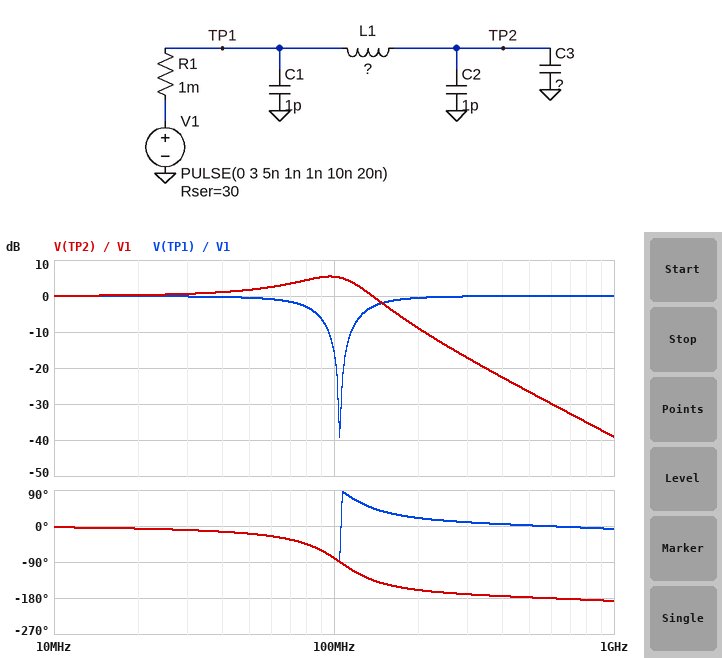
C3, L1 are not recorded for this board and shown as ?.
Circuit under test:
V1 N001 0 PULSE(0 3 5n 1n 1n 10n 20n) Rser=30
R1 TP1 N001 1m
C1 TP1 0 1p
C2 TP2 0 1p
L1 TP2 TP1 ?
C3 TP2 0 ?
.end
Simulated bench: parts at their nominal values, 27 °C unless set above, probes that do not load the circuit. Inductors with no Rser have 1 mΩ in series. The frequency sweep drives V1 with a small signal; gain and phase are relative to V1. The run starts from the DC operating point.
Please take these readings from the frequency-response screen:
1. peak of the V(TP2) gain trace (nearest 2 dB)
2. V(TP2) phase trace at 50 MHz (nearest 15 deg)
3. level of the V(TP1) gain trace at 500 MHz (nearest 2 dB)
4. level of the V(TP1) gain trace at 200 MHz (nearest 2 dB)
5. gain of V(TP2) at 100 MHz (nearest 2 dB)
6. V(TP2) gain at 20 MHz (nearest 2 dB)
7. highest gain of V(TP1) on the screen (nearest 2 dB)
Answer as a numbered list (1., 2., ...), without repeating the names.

1. 6 dB
2. -15 deg
3. 0 dB
4. 0 dB
5. 6 dB
6. 0 dB
7. 0 dB
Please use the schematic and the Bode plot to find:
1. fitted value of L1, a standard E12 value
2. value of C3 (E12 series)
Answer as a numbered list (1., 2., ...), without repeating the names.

1. 82 nH
2. 27 pF
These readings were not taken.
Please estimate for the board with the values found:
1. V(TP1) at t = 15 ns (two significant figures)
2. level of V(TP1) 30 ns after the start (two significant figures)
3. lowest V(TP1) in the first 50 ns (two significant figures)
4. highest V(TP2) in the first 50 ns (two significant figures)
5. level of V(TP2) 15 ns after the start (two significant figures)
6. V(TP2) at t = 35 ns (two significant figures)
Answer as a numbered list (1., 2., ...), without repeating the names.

1. 3.1 V
2. 2.9 V
3. -410 mV
4. 4.2 V
5. 2.5 V
6. 2.6 V
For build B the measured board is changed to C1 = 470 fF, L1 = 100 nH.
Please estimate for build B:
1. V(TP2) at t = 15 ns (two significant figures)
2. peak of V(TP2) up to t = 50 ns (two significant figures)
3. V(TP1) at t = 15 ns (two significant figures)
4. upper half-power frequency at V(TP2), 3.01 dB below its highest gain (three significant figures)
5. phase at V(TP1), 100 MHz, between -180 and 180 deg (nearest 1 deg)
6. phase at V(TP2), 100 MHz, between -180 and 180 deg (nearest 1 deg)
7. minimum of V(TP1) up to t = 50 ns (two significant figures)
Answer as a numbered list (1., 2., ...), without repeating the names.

1. 2.6 V
2. 4.3 V
3. 3.3 V
4. 111 MHz
5. 79 deg
6. -101 deg
7. -380 mV
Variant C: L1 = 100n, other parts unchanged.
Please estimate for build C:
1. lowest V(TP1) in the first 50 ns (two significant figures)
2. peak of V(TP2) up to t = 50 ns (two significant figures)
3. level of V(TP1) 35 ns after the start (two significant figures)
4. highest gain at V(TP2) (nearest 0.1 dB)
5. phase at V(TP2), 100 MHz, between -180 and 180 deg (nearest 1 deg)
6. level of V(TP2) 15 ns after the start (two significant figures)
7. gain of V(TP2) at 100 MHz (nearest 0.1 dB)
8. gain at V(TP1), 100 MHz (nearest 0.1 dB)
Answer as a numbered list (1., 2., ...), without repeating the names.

1. -380 mV
2. 4.3 V
3. 3.2 V
4. 6.2 dB
5. -101 deg
6. 2.6 V
7. 5.4 dB
8. -14.1 dB
